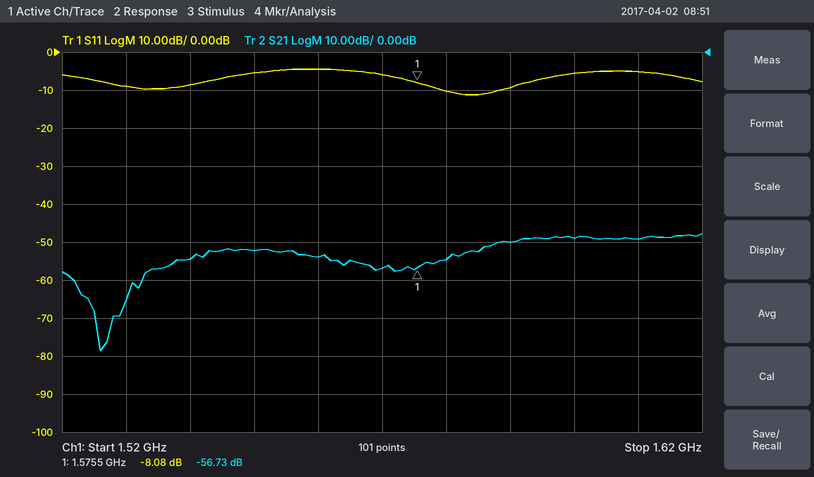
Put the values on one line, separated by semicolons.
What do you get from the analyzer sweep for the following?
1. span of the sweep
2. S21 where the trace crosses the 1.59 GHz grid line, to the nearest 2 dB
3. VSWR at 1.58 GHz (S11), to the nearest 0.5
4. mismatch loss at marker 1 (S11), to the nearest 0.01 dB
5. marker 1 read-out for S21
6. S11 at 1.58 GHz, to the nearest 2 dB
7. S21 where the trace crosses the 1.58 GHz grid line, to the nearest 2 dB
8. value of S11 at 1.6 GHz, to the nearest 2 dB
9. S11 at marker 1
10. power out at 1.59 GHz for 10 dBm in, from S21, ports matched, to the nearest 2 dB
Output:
100 MHz; -50 dB; 2.0; 0.73 dB; -56.73 dB; -10 dB; -54 dB; -6 dB; -8.08 dB; -40 dBm
